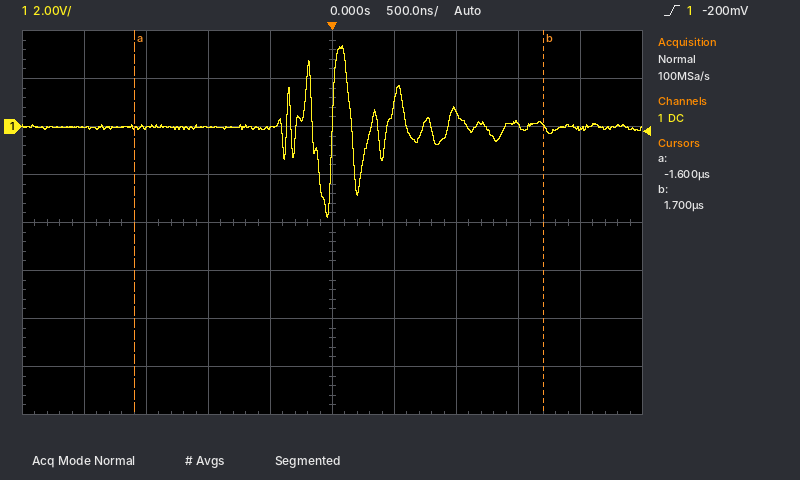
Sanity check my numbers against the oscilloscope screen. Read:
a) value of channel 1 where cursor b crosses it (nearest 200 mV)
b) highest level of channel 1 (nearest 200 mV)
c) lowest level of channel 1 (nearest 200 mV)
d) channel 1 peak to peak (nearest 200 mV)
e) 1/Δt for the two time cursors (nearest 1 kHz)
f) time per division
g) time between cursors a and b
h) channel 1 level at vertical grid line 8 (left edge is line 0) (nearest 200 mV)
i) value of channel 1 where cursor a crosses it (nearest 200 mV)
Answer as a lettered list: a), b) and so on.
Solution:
a) 0.0 V
b) 3.4 V
c) -3.8 V
d) 7.2 V
e) 303 kHz
f) 500 ns
g) 3.30 µs
h) 0.0 V
i) 0.0 V
